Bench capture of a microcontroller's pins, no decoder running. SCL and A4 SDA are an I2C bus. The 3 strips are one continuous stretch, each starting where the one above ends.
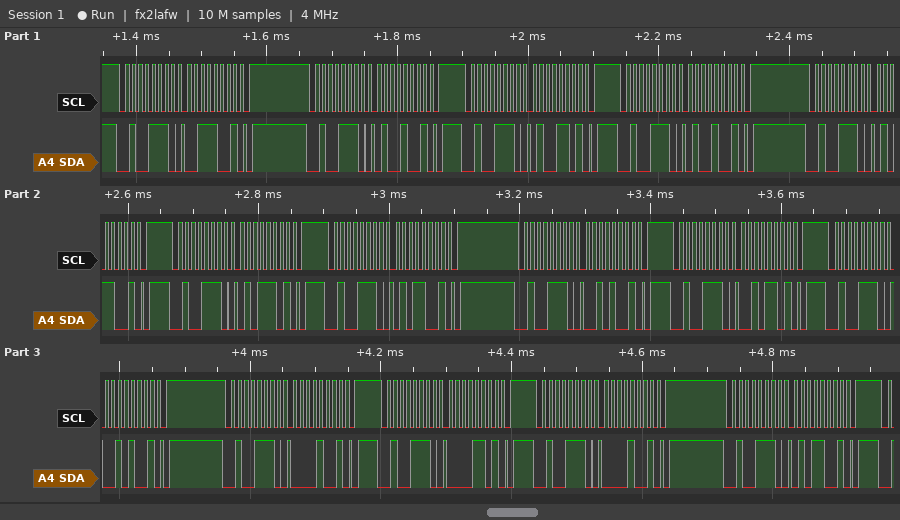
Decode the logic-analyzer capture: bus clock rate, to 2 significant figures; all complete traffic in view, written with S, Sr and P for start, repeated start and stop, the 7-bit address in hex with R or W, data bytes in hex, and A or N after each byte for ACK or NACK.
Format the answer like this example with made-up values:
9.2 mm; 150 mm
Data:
100 kHz; S 27W A 39 A P S 27W A 49 A P S 27W A 4D A P S 27W A 49 A P S 27W A 59 A P S 27W A 5D A P S 27W A 59 A P S 27W A 29 A P S 27W A 2D A P S 27W A 29 A P S 27W A 09 A P S 27W A 0D A P S 27W A 09 A P S 27W A 59 A P
